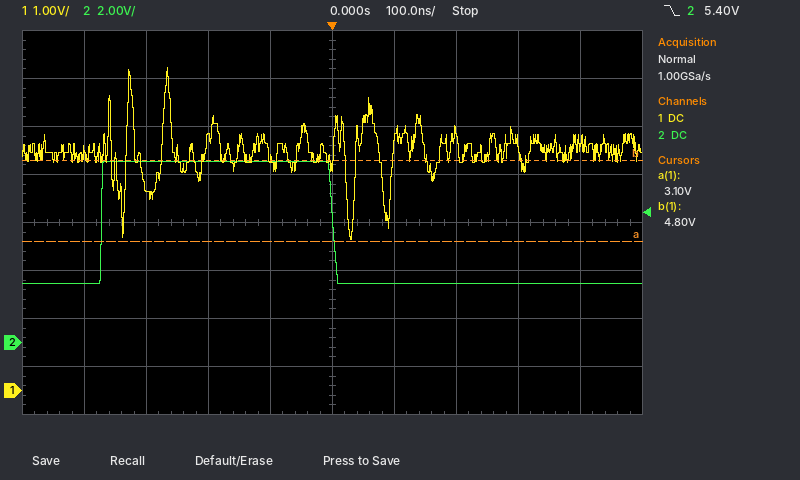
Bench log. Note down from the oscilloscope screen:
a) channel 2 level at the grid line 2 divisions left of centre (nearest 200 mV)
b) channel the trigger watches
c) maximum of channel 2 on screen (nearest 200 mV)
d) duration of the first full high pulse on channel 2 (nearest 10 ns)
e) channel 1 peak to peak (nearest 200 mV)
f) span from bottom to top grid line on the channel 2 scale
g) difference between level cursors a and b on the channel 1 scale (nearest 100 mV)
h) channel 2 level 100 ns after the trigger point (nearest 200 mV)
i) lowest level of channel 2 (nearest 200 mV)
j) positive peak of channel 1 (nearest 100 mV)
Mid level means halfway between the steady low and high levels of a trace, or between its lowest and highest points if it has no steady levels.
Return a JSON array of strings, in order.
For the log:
["7.6 V", "channel 2", "7.6 V", "370 ns", "3.6 V", "16 V", "1.7 V", "2.4 V", "2.4 V", "6.7 V"]
